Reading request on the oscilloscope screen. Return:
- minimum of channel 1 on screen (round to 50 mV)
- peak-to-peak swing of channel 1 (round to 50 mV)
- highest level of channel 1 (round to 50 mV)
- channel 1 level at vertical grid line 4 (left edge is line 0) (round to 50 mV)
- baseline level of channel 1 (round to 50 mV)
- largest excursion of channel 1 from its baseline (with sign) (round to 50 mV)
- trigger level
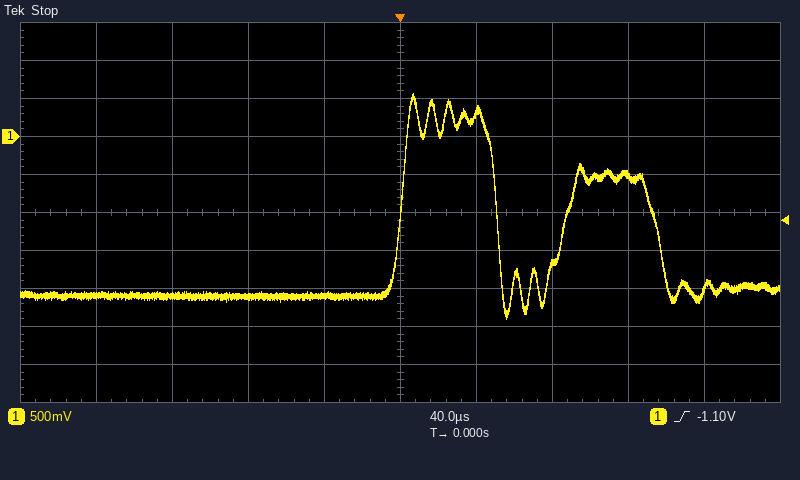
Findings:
-2.40 V
2.95 V
550 mV
-2.10 V
-2.10 V
+2.65 V
-1.10 V
